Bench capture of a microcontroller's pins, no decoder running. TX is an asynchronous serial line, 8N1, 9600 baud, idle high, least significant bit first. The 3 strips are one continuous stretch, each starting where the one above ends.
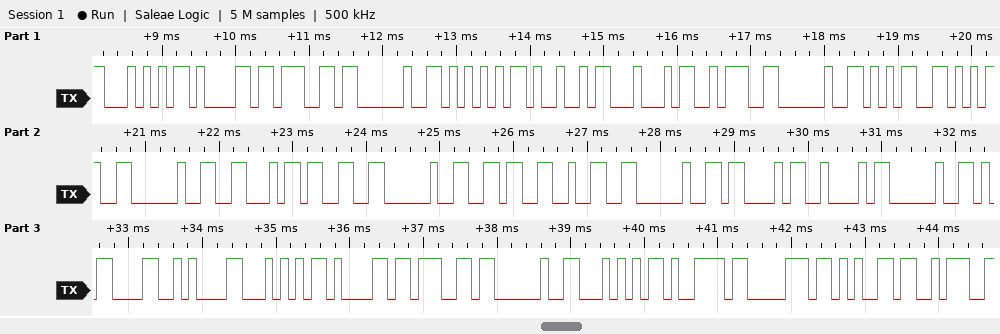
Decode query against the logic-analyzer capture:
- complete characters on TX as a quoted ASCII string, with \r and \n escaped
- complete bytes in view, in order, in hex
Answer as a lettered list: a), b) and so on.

a) "Tag UID: 55 F3 62 CB \r\nTag Type:"
b) 0x54 0x61 0x67 0x20 0x55 0x49 0x44 0x3A 0x20 0x35 0x35 0x20 0x46 0x33 0x20 0x36 0x32 0x20 0x43 0x42 0x20 0x0D 0x0A 0x54 0x61 0x67 0x20 0x54 0x79 0x70 0x65 0x3A
